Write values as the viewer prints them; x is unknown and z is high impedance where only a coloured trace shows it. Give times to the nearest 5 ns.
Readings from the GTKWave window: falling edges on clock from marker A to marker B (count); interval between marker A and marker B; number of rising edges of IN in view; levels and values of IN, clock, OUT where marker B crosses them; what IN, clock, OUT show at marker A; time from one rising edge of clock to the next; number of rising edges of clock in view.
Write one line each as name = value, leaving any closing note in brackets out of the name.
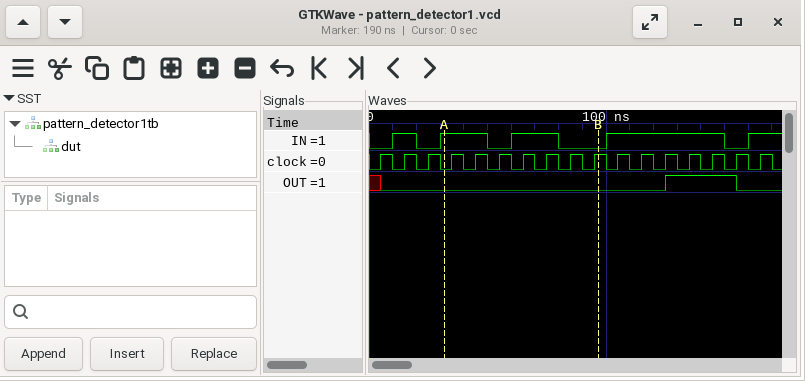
falling edges on clock from marker A to marker B = 6
interval between marker A and marker B = 65 ns
number of rising edges of IN in view = 5
levels and values of IN, clock, OUT where marker B crosses them = IN=0, clock=1, OUT=0
what IN, clock, OUT show at marker A = IN=1, clock=0, OUT=0
time from one rising edge of clock to the next = 10 ns
number of rising edges of clock in view = 17
